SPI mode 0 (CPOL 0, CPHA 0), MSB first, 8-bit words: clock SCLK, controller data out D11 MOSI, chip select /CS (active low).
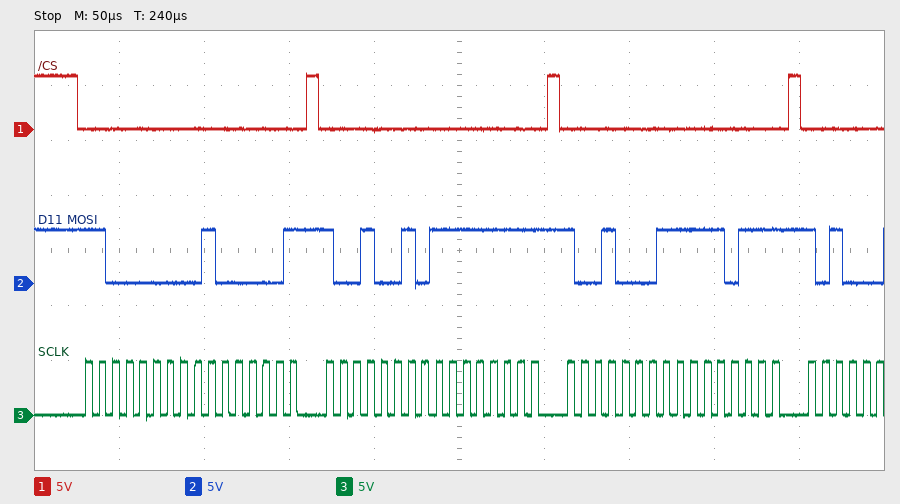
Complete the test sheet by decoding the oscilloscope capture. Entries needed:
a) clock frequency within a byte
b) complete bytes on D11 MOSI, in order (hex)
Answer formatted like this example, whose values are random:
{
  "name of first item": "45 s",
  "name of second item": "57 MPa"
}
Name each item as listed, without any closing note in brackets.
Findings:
{
  "clock frequency within a byte": "125 kHz",
  "complete bytes on D11 MOSI, in order": "0xC0 0x41 0x92 0xFF 0x91 0xF7"
}
